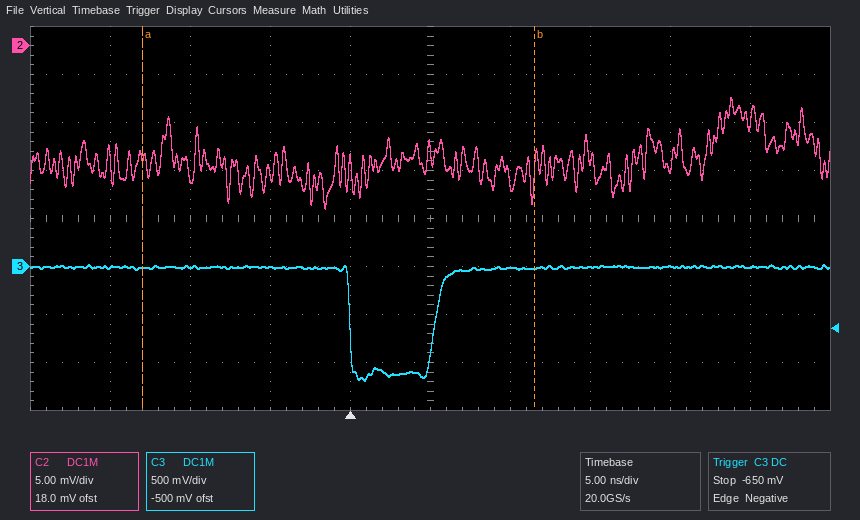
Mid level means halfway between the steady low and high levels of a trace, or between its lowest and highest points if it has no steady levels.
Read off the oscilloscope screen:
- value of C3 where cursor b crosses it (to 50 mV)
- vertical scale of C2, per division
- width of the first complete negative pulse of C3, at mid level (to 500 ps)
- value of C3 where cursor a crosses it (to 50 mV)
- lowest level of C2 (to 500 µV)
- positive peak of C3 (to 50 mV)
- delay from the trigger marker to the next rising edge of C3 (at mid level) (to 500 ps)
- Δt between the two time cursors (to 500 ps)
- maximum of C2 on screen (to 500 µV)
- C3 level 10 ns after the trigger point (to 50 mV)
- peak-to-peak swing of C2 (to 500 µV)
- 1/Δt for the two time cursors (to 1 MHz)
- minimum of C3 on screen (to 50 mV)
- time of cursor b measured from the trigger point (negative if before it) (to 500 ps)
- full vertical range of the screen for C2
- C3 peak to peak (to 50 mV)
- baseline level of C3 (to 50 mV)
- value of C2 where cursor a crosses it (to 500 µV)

0 mV
5 mV
5.5 ns
0 mV
-17.0 mV
0 mV
5.5 ns
24.5 ns
-5.5 mV
0 mV
11.5 mV
41 MHz
-1.20 V
+11.5 ns
40 mV
1.20 V
0 mV
-11.5 mV
